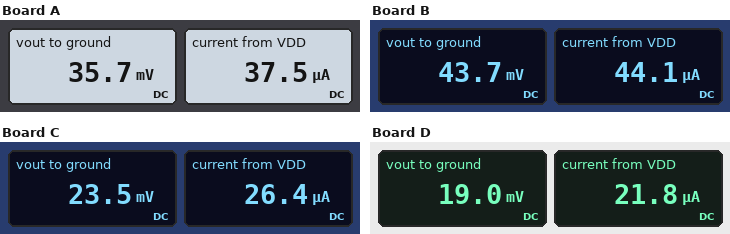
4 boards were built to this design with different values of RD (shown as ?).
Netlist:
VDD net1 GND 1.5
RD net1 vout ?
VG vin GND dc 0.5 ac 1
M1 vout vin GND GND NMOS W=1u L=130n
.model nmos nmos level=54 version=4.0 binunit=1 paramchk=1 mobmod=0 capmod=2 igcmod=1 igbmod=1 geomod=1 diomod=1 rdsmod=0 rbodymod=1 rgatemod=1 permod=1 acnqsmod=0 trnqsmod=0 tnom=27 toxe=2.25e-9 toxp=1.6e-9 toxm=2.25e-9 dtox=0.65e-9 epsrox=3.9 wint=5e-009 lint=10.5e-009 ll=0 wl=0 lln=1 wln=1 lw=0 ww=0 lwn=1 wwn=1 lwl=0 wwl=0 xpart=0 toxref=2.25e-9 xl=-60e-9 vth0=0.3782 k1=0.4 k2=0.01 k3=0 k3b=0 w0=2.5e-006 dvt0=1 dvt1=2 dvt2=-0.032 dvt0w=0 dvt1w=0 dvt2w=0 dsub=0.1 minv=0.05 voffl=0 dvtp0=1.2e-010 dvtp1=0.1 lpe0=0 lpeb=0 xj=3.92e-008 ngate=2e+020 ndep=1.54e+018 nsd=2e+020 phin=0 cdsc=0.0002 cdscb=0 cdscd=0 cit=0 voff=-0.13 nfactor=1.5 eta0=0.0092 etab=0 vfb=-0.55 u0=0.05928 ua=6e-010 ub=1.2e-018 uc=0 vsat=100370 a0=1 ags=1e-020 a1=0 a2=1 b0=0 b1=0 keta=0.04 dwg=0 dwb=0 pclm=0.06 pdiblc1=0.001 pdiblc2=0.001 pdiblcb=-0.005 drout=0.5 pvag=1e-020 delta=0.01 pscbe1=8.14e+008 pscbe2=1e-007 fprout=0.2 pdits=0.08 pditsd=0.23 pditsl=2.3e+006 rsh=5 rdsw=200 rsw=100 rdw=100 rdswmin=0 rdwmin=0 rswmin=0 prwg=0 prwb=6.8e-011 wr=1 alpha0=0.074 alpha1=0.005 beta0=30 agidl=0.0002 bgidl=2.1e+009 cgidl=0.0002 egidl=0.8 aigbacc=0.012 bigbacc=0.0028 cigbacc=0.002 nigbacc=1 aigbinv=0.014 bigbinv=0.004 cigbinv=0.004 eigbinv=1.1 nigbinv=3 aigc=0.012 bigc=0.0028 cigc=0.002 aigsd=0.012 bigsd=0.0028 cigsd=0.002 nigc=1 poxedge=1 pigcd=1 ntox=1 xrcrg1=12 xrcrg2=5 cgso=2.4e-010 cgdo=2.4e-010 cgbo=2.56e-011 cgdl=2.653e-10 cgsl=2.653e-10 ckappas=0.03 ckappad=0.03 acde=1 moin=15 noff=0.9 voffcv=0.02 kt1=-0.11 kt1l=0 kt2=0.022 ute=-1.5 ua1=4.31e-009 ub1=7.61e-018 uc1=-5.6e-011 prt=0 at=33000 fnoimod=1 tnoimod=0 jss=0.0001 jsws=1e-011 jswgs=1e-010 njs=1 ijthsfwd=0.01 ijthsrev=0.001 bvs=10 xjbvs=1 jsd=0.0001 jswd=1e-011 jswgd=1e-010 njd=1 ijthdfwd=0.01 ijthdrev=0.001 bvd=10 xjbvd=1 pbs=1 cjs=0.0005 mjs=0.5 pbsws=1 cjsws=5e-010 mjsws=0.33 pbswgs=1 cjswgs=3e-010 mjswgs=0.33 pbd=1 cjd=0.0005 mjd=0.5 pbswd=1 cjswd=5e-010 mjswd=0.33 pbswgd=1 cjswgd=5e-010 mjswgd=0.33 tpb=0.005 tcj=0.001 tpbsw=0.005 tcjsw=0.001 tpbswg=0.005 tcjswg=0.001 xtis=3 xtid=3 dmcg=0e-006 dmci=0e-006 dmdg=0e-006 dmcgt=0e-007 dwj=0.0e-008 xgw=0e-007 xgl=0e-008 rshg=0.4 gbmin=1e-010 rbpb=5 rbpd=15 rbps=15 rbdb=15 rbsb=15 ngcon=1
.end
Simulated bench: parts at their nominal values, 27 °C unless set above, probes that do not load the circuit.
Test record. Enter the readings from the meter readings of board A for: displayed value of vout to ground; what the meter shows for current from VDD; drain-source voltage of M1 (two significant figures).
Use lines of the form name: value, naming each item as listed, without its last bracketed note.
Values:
displayed value of vout to ground: 35.7 mV
what the meter shows for current from VDD: 37.5 µA
drain-source voltage of M1: 36 mV
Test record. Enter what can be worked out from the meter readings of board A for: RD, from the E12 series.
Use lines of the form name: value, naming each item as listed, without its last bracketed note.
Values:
RD, from the E12 series: 39 kΩ
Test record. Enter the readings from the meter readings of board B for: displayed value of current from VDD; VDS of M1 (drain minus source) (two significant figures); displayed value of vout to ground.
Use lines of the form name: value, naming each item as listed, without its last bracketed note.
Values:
displayed value of current from VDD: 44.1 µA
VDS of M1 (drain minus source): 44 mV
displayed value of vout to ground: 43.7 mV
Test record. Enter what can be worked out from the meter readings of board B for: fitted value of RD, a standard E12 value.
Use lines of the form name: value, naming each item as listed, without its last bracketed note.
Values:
fitted value of RD, a standard E12 value: 33 kΩ
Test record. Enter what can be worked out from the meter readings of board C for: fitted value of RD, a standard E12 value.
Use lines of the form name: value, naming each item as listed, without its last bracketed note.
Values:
fitted value of RD, a standard E12 value: 56 kΩ
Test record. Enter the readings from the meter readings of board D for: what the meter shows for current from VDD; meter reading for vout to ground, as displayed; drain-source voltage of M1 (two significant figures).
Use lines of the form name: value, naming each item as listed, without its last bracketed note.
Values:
what the meter shows for current from VDD: 21.8 µA
meter reading for vout to ground, as displayed: 19.0 mV
drain-source voltage of M1: 19 mV
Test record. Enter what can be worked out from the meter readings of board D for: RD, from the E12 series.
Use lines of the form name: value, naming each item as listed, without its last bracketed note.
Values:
RD, from the E12 series: 68 kΩ
